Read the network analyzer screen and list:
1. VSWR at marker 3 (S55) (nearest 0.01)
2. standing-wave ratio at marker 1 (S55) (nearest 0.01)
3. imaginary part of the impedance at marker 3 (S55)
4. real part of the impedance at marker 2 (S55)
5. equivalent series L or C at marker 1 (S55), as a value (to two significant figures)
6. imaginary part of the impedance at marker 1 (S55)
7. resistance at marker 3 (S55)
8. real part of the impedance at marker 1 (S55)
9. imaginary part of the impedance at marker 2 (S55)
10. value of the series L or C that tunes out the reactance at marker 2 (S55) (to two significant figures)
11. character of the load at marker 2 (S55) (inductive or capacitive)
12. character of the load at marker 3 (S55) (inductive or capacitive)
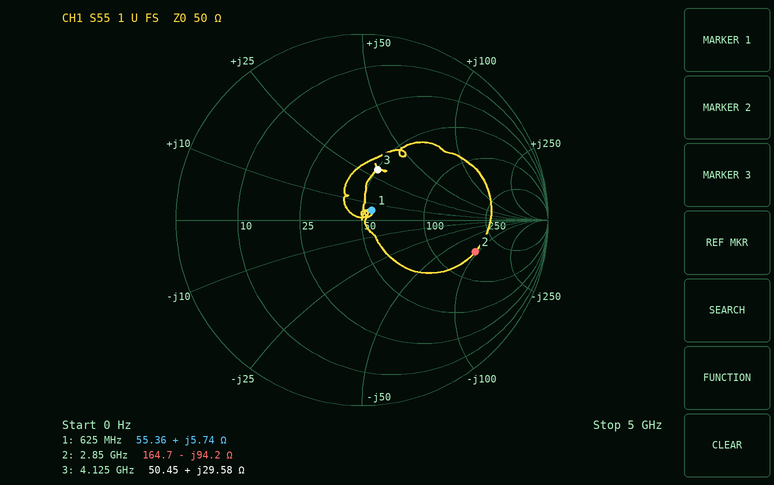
1.79
1.16
+29.58 Ω
164.7 Ω
1.5 nH
+5.74 Ω
50.45 Ω
55.36 Ω
-94.2 Ω
5.3 nH
capacitive
inductive
